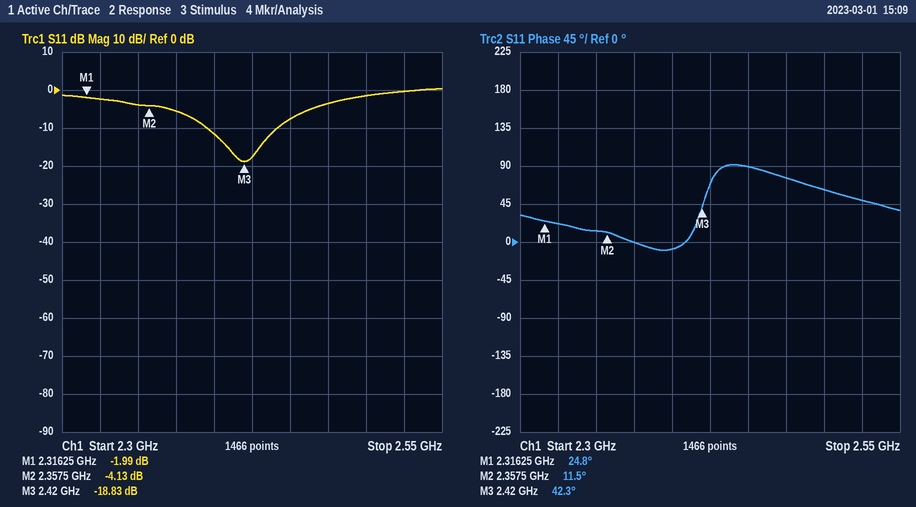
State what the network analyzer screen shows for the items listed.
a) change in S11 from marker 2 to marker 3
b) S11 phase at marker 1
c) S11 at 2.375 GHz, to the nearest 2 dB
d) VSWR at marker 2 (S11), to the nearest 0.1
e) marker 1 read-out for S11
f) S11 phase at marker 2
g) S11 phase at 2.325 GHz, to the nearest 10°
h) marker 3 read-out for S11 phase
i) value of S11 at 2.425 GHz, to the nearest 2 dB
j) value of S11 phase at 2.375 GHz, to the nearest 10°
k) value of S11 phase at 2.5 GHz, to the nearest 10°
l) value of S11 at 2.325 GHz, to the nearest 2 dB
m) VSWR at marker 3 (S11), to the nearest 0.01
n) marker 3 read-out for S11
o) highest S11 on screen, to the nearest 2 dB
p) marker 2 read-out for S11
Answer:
-14.70 dB
24.8°
-6 dB
4.3
-1.99 dB
11.5°
20°
42.3°
-18 dB
0°
60°
-2 dB
1.26
-18.83 dB
0 dB
-4.13 dB
